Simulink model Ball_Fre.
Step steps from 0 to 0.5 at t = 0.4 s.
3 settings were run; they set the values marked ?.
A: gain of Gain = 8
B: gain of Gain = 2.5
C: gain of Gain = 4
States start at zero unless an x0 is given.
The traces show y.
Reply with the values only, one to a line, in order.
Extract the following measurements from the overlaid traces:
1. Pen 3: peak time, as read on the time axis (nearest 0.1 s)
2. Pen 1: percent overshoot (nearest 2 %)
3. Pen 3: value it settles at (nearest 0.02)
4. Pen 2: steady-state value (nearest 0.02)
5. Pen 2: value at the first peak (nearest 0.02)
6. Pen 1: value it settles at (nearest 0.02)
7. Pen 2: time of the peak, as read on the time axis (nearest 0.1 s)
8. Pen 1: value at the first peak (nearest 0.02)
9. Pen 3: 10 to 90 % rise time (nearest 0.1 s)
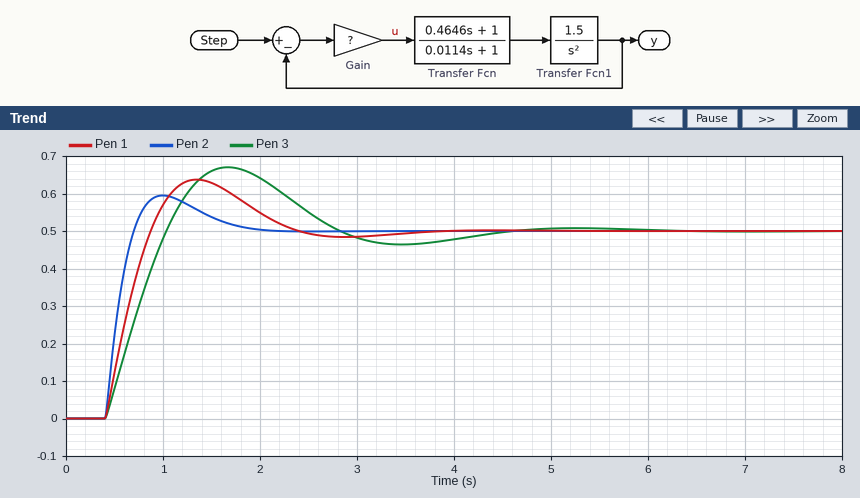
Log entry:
1.7 s
28 %
0.50
0.50
0.60
0.50
1.0 s
0.64
0.5 s
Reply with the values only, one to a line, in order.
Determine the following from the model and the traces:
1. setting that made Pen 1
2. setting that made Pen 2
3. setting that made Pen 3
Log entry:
C
A
B
